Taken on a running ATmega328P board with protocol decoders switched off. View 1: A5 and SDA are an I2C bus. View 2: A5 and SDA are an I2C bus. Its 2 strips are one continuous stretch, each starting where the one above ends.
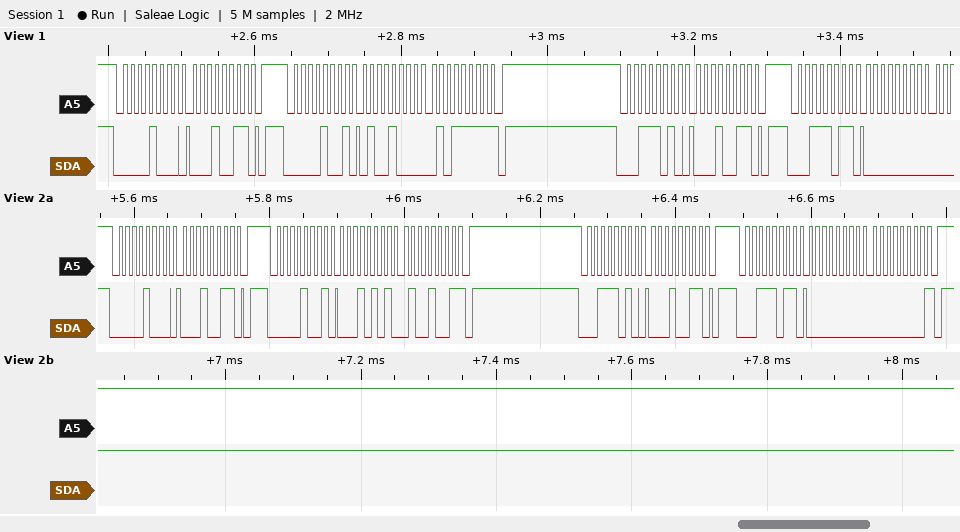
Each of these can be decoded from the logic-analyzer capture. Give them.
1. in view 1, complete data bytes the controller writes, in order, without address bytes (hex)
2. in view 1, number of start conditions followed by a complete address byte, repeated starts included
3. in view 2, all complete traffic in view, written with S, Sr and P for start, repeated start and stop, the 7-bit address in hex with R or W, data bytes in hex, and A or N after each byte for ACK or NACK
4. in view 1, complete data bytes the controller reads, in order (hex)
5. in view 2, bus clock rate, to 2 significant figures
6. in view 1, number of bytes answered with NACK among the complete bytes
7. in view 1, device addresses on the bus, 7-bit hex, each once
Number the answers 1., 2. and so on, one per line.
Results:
1. 13 13
2. 4
3. S 04W A 13 A P S 04R A 15 A 49 N P S 1DW A 13 A P S 1DR A 00 A 00 N P
4. 48 5F 00
5. 100 kHz
6. 1
7. 0x04 0x1D
